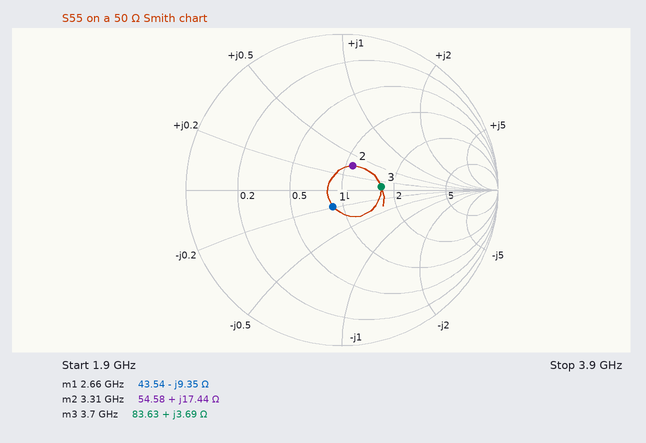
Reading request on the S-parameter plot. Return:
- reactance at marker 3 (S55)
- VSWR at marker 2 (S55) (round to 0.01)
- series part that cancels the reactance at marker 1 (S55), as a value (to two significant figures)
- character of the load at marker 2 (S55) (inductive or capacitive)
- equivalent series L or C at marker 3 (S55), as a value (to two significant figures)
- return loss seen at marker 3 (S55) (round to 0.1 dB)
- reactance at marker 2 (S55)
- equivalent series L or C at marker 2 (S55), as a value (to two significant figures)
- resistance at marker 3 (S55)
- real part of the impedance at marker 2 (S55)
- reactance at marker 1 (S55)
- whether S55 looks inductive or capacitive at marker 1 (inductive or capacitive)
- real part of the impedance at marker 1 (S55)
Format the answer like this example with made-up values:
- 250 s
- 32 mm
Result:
- +3.69 Ω
- 1.41
- 560 pH
- inductive
- 160 pH
- 11.9 dB
- +17.44 Ω
- 840 pH
- 83.63 Ω
- 54.58 Ω
- -9.35 Ω
- capacitive
- 43.54 Ω
